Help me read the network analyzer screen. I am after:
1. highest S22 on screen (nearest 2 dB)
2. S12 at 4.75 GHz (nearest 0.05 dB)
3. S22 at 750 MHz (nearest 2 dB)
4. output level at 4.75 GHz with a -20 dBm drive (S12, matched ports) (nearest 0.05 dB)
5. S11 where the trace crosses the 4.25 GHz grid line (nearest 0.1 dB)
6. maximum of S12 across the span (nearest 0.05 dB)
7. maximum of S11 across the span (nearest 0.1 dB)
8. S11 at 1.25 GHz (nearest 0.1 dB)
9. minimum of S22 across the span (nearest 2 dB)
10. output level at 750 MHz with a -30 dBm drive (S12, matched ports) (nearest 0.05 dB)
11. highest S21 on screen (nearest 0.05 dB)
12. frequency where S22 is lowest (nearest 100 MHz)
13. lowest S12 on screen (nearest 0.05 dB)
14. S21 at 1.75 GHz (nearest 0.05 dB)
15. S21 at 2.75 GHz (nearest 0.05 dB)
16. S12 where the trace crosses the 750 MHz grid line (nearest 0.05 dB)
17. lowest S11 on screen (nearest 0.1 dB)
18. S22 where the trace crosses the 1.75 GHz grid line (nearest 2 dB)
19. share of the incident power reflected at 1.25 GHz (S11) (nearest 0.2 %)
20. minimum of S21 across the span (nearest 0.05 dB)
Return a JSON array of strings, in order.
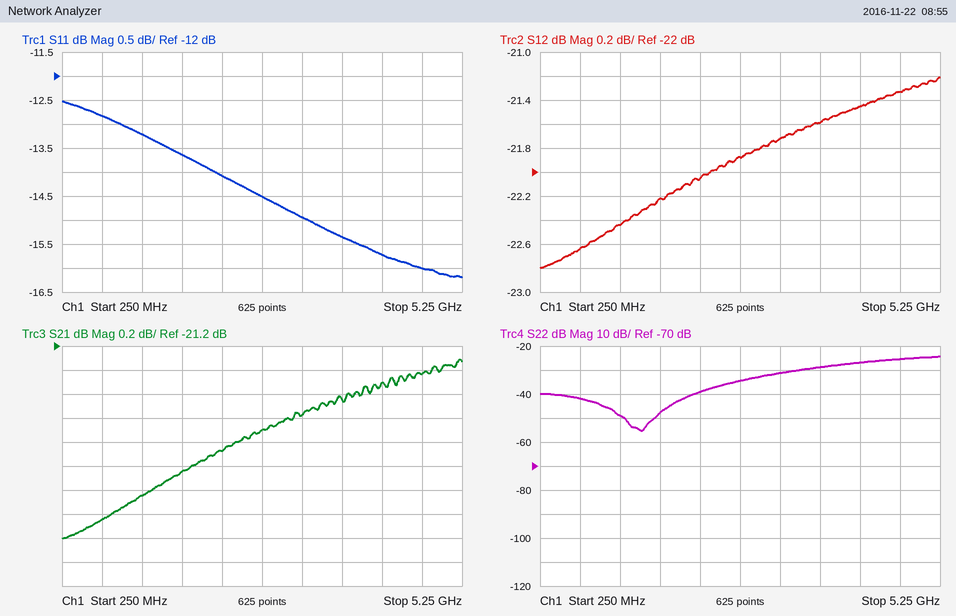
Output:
["-24 dB", "-21.35 dB", "-42 dB", "-41.35 dBm", "-15.7 dB", "-21.20 dB", "-12.5 dB", "-13.2 dB", "-56 dB", "-52.65 dBm", "-21.30 dB", "1.5 GHz", "-22.80 dB", "-22.25 dB", "-21.90 dB", "-22.65 dB", "-16.2 dB", "-48 dB", "4.8 %", "-22.80 dB"]
